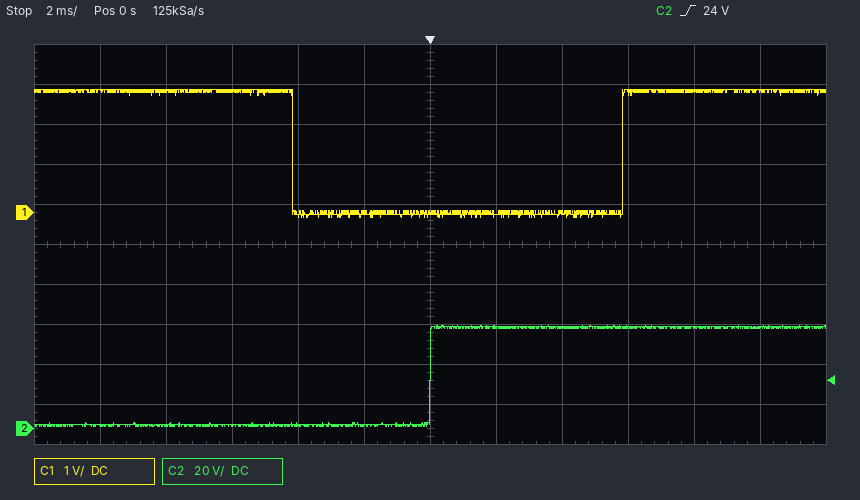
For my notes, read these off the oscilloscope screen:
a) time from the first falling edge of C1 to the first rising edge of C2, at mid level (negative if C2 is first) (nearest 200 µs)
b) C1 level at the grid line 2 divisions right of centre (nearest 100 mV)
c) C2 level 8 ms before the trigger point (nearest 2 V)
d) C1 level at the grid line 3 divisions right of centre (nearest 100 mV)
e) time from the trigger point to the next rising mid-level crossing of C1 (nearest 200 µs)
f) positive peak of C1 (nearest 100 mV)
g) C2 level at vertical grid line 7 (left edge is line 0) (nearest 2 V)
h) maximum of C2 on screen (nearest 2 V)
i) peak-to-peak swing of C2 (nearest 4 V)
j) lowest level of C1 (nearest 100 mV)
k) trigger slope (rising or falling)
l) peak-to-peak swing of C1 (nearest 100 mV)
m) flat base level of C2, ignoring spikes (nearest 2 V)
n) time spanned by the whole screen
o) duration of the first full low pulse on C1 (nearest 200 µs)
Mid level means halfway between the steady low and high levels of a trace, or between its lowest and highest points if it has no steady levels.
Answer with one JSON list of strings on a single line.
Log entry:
["+4.2 ms", "0.0 V", "2 V", "3.0 V", "5.8 ms", "3.1 V", "50 V", "52 V", "52 V", "-100 mV", "rising", "3.2 V", "2 V", "24 ms", "10.0 ms"]
